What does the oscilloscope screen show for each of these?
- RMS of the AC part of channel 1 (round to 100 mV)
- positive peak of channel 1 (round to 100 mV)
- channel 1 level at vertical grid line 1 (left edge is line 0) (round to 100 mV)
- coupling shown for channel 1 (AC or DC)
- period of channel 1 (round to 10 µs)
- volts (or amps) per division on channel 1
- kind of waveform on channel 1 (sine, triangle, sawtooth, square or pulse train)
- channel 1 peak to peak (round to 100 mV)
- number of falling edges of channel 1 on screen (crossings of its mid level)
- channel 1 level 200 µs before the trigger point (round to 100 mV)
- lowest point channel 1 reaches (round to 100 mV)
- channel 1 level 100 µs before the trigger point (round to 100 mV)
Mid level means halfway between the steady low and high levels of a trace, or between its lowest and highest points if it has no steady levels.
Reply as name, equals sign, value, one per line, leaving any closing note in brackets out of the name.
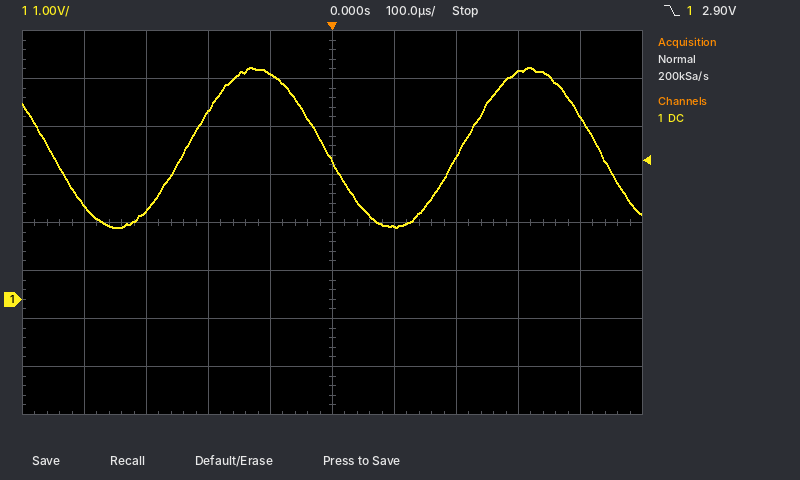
RMS of the AC part of channel 1 = 1.2 V
positive peak of channel 1 = 4.8 V
channel 1 level at vertical grid line 1 (left edge is line 0) = 2.0 V
coupling shown for channel 1 = DC
period of channel 1 = 440 µs
volts (or amps) per division on channel 1 = 1 V
kind of waveform on channel 1 = sine
channel 1 peak to peak = 3.3 V
number of falling edges of channel 1 on screen = 3
channel 1 level 200 µs before the trigger point = 3.9 V
lowest point channel 1 reaches = 1.5 V
channel 1 level 100 µs before the trigger point = 4.7 V
